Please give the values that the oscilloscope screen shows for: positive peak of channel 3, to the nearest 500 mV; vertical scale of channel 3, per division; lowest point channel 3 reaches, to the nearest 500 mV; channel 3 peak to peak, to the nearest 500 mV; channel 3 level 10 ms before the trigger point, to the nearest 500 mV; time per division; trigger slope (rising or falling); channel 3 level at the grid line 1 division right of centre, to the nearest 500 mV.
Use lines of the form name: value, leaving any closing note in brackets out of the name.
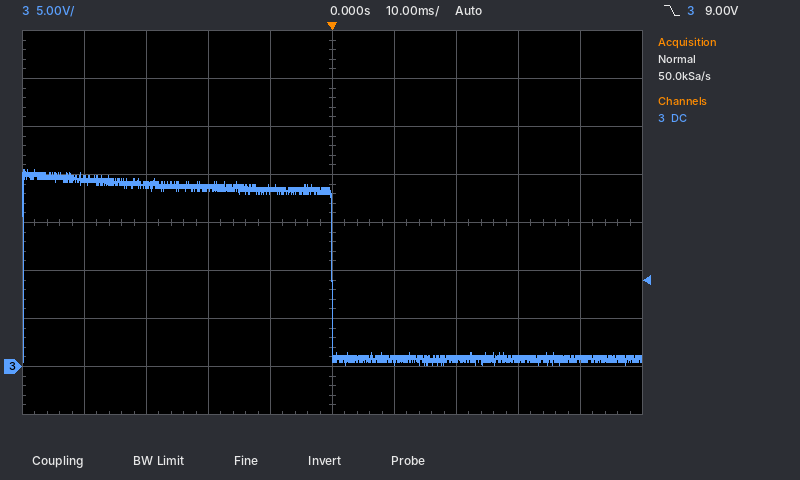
positive peak of channel 3, to the nearest 500 mV: 20.5 V
vertical scale of channel 3, per division: 5 V
lowest point channel 3 reaches, to the nearest 500 mV: 0.0 V
channel 3 peak to peak, to the nearest 500 mV: 20.5 V
channel 3 level 10 ms before the trigger point, to the nearest 500 mV: 18.5 V
time per division: 10 ms
trigger slope: falling
channel 3 level at the grid line 1 division right of centre, to the nearest 500 mV: 500 mV
